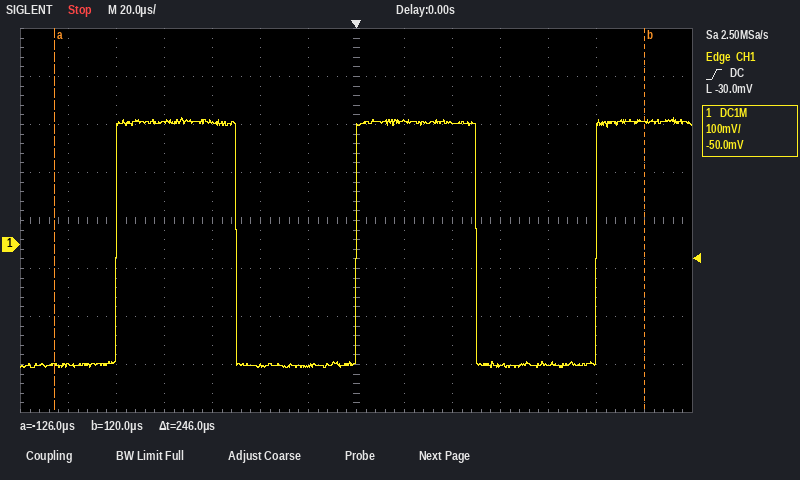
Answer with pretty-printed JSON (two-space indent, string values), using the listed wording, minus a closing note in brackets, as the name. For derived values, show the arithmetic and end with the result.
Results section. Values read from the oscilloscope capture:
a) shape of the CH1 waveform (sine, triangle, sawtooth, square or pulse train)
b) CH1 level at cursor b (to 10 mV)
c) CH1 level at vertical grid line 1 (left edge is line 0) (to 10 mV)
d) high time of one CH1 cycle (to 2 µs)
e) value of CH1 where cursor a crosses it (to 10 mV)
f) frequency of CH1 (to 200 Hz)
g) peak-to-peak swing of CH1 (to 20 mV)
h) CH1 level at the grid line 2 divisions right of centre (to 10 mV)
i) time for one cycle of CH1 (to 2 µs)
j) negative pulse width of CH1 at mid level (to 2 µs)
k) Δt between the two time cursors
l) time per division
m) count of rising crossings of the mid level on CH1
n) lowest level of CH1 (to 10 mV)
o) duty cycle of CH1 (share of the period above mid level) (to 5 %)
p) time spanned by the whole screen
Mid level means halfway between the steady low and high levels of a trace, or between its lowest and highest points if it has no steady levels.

{
  "shape of the CH1 waveform": "square",
  "CH1 level at cursor b": "260 mV",
  "CH1 level at vertical grid line 1 (left edge is line 0)": "-250 mV",
  "high time of one CH1 cycle": "50 µs",
  "value of CH1 where cursor a crosses it": "-250 mV",
  "frequency of CH1": "1 / 100 µs ≈ 10.0 kHz",
  "peak-to-peak swing of CH1": "520 mV",
  "CH1 level at the grid line 2 divisions right of centre": "250 mV",
  "time for one cycle of CH1": "100 µs",
  "negative pulse width of CH1 at mid level": "50 µs",
  "Δt between the two time cursors": "246 µs",
  "time per division": "20 µs",
  "count of rising crossings of the mid level on CH1": "3",
  "lowest level of CH1": "-260 mV",
  "duty cycle of CH1 (share of the period above mid level)": "50 µs / 100 µs ≈ 50 %",
  "time spanned by the whole screen": "280 µs"
}
